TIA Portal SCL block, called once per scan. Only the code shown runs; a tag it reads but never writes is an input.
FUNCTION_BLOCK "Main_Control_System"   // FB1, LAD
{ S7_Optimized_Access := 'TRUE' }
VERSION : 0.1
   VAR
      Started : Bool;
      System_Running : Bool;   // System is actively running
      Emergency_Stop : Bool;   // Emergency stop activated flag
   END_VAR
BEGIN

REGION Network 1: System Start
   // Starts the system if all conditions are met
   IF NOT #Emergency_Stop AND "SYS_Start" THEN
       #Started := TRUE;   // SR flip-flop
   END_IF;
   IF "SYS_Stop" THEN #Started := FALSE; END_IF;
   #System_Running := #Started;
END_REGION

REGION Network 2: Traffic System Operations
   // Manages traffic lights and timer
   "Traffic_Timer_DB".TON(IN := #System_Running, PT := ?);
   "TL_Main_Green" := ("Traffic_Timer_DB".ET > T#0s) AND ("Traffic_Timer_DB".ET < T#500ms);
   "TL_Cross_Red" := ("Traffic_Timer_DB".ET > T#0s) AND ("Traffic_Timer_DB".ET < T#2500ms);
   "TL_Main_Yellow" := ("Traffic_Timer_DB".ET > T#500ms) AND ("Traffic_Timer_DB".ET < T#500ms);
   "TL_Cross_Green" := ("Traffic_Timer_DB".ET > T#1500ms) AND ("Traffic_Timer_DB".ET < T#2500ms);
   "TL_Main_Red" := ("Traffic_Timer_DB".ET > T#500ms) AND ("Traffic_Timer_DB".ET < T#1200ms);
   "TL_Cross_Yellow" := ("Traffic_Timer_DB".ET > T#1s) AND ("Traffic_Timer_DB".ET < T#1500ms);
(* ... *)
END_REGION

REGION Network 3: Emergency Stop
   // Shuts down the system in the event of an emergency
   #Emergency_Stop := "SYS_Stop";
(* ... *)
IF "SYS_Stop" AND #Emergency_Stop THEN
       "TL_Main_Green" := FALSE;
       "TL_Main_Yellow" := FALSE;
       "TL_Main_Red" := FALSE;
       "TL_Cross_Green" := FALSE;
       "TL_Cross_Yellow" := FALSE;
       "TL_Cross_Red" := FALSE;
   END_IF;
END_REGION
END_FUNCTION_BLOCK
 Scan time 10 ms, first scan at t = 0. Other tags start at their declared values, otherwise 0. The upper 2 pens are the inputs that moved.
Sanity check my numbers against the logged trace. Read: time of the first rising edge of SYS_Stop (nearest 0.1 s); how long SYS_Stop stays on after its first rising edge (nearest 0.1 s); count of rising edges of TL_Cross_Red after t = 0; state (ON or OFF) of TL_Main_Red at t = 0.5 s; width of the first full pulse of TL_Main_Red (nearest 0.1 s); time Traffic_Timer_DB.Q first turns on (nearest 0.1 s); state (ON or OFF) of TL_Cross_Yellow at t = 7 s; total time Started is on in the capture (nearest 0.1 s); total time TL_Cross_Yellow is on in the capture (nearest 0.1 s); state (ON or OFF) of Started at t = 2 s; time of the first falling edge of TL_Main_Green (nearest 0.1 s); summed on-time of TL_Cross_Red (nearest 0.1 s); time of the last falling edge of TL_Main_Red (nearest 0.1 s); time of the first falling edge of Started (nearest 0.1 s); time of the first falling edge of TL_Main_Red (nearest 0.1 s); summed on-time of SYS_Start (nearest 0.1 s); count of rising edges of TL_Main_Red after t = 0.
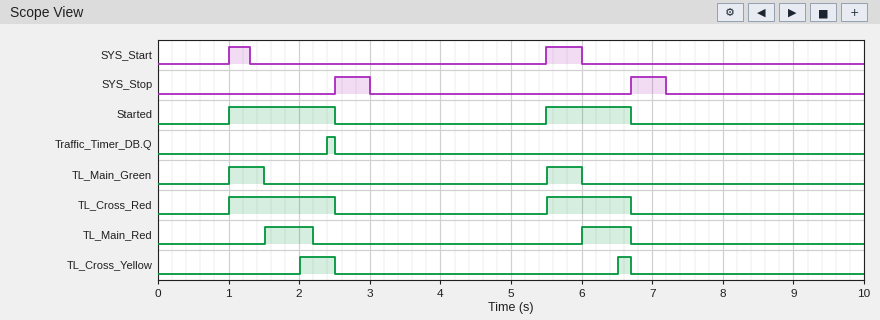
2.5 s
0.5 s
2
OFF
0.7 s
2.4 s
OFF
2.7 s
0.7 s
ON
1.5 s
2.7 s
6.7 s
2.5 s
2.2 s
0.8 s
2
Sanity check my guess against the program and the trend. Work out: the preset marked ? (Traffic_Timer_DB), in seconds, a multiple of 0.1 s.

1.4 s
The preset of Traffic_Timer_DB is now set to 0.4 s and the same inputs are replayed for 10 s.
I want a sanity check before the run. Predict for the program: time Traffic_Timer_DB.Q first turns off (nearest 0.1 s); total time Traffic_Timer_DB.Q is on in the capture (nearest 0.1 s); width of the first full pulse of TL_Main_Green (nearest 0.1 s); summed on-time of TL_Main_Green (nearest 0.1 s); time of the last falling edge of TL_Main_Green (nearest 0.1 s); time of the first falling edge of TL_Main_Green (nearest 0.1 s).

2.5 s
1.9 s
1.5 s
2.7 s
6.7 s
2.5 s
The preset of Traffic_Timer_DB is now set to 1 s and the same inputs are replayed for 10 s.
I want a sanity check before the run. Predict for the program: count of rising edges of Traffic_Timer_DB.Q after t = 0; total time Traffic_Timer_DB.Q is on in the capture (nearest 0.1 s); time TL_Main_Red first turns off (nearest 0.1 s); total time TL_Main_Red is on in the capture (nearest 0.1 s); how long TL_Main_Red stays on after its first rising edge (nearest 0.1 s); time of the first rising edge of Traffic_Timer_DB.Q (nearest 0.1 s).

2
0.7 s
2.5 s
1.7 s
1.0 s
2.0 s
